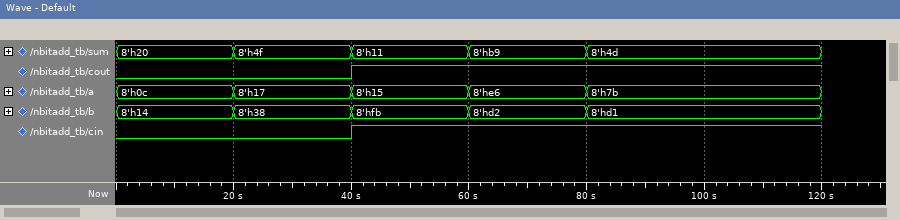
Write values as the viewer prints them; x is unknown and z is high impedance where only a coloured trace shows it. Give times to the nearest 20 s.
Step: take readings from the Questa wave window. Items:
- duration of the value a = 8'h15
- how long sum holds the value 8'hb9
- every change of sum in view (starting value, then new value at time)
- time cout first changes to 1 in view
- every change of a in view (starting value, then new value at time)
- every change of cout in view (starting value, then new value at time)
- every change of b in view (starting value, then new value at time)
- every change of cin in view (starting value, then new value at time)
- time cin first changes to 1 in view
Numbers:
20 s
20 s
8'h20, 8'h4f at 20 s, 8'h11 at 40 s, 8'hb9 at 60 s, 8'h4d at 80 s
40 s
8'h0c, 8'h17 at 20 s, 8'h15 at 40 s, 8'he6 at 60 s, 8'h7b at 80 s
0, 1 at 40 s
8'h14, 8'h38 at 20 s, 8'hfb at 40 s, 8'hd2 at 60 s, 8'hd1 at 80 s
0, 1 at 40 s
40 s
